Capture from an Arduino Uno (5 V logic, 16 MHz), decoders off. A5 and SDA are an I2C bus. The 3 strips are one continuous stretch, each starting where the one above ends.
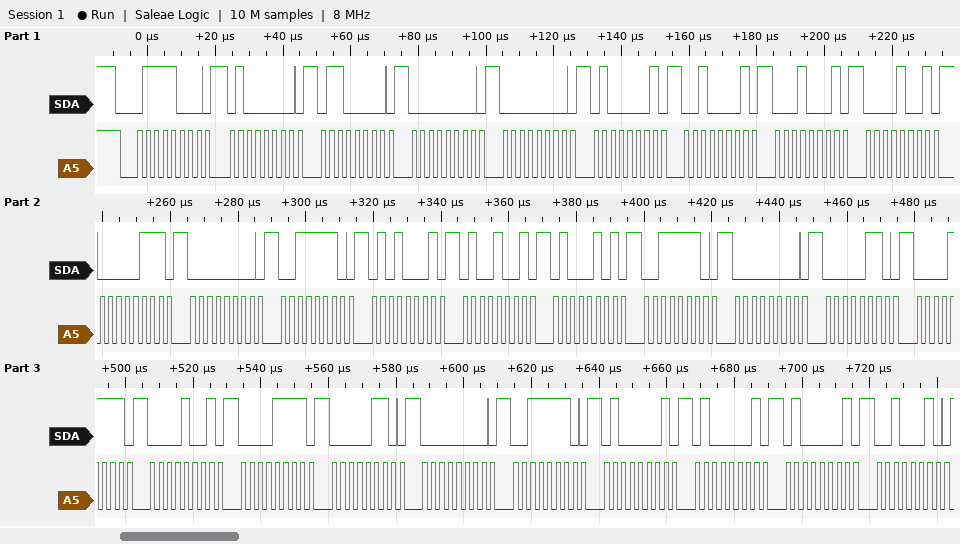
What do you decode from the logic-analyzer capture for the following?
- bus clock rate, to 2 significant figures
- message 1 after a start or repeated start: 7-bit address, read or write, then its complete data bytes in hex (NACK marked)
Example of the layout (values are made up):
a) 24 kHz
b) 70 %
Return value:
a) 400 kHz
b) 0x3C write: 40 60 00 00 41 21 11 09 07 00 3E 51 49 45 3E 00 06 0F 09 0F 06 00 3E 41 41 41 22
